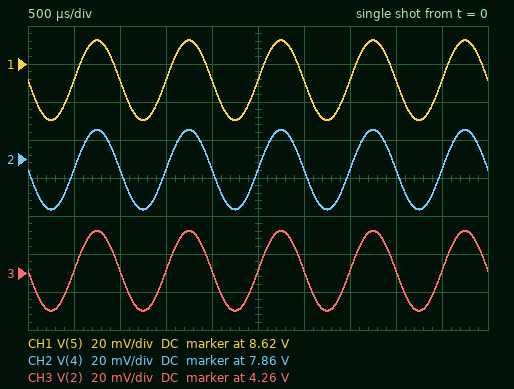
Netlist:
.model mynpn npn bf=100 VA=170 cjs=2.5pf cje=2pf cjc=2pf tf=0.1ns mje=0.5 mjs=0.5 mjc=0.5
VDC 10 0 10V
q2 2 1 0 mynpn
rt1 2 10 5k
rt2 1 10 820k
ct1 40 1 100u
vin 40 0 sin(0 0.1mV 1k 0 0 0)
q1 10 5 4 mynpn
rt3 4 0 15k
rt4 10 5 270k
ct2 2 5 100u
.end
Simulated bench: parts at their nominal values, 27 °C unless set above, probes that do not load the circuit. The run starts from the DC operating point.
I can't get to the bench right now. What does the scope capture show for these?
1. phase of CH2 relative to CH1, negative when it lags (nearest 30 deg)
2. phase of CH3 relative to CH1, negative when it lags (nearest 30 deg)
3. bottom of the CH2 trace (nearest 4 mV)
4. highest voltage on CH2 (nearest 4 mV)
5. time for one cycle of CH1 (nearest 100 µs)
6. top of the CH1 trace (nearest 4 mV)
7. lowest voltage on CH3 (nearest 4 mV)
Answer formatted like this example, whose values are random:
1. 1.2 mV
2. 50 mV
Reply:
1. 0 deg
2. 0 deg
3. 7.832 V
4. 7.876 V
5. 1.0 ms
6. 8.632 V
7. 4.240 V
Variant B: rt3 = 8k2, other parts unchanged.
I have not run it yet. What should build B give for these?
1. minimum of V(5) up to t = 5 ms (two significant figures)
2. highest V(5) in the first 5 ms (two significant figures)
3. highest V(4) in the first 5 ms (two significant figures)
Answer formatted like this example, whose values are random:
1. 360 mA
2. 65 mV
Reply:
1. 7.7 V
2. 7.8 V
3. 7.0 V
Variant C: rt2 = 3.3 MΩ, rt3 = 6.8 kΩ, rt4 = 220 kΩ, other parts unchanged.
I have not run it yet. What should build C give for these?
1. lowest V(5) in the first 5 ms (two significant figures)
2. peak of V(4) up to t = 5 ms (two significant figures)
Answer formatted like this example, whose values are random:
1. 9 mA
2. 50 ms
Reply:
1. 7.8 V
2. 7.0 V
